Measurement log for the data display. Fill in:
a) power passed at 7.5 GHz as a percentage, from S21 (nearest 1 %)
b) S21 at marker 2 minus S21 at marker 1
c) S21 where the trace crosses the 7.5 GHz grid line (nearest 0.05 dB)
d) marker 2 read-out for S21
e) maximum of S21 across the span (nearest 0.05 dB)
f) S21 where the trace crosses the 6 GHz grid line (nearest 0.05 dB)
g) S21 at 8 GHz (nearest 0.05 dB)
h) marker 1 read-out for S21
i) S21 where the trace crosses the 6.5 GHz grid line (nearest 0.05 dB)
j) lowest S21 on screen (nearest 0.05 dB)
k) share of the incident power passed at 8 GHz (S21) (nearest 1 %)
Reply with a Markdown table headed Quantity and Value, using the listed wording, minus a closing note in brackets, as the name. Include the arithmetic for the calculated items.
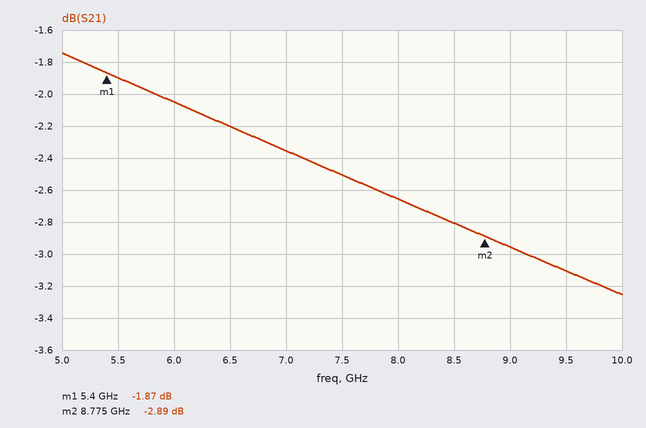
| Quantity | Value |
|---|---|
| power passed at 7.5 GHz as a percentage, from S21 | 10^(-2.5/10) ≈ 56 % |
| S21 at marker 2 minus S21 at marker 1 | -2.89 − (-1.87) = -1.02 dB |
| S21 where the trace crosses the 7.5 GHz grid line | -2.50 dB |
| marker 2 read-out for S21 | -2.89 dB |
| maximum of S21 across the span | -1.75 dB |
| S21 where the trace crosses the 6 GHz grid line | -2.05 dB |
| S21 at 8 GHz | -2.65 dB |
| marker 1 read-out for S21 | -1.87 dB |
| S21 where the trace crosses the 6.5 GHz grid line | -2.20 dB |
| lowest S21 on screen | -3.25 dB |
| share of the incident power passed at 8 GHz (S21) | 10^(-2.65/10) ≈ 54 % |
